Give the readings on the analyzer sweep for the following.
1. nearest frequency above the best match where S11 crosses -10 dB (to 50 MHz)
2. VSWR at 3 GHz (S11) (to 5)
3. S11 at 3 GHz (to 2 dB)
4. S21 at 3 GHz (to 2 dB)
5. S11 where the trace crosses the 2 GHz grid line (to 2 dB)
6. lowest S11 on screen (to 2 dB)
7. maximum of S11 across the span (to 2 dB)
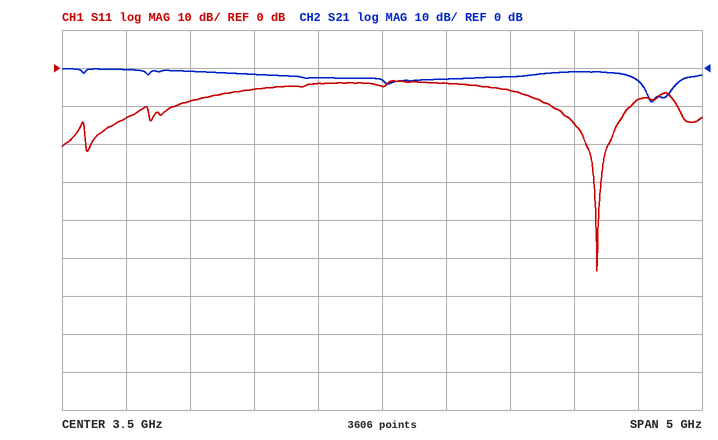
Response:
5.45 GHz
5
-4 dB
-2 dB
-8 dB
-54 dB
-4 dB
